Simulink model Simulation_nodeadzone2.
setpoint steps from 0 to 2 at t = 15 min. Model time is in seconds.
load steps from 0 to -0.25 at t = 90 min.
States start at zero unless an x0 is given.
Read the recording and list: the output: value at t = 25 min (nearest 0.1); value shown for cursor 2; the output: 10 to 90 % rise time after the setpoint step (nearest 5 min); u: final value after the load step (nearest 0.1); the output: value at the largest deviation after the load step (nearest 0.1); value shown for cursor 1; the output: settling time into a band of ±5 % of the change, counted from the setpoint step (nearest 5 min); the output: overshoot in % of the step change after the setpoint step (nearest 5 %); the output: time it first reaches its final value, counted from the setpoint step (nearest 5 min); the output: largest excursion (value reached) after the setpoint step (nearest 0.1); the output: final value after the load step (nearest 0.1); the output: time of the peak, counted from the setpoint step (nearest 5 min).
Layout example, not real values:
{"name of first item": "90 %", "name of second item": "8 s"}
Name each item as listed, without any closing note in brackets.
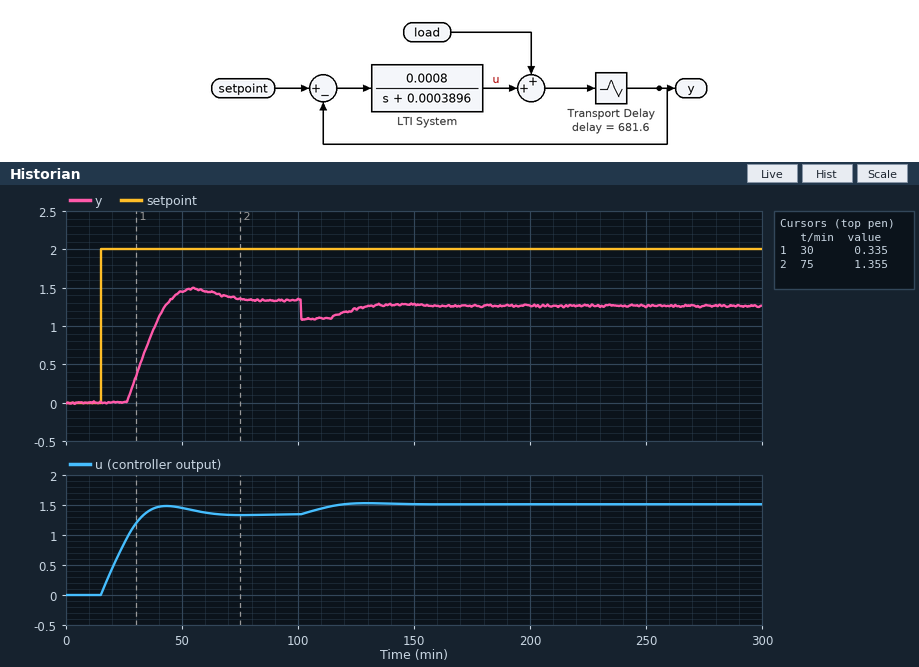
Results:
{"the output: value at t = 25 min": "0.0", "value shown for cursor 2": "1.355", "the output: 10 to 90 % rise time after the setpoint step": "15 min", "u: final value after the load step": "1.5", "the output: value at the largest deviation after the load step": "1.1", "value shown for cursor 1": "0.335", "the output: settling time into a band of ±5 % of the change, counted from the setpoint step": "50 min", "the output: overshoot in % of the step change after the setpoint step": "10 %", "the output: time it first reaches its final value, counted from the setpoint step": "30 min", "the output: largest excursion (value reached) after the setpoint step": "1.5", "the output: final value after the load step": "1.3", "the output: time of the peak, counted from the setpoint step": "40 min"}
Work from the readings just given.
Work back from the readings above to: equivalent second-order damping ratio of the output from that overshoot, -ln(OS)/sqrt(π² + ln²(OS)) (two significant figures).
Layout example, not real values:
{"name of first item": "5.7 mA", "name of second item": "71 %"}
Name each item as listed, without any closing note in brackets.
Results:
{"equivalent second-order damping ratio of the output from that overshoot, -ln(OS)/sqrt(π² + ln²(OS))": "0.59"}
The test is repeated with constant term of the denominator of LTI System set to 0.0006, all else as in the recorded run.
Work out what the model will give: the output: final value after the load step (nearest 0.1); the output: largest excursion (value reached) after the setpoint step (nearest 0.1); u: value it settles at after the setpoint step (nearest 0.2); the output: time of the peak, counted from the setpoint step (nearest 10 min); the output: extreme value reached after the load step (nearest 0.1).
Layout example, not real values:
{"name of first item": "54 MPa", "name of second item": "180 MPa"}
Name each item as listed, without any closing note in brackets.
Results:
{"the output: final value after the load step": "1.0", "the output: largest excursion (value reached) after the setpoint step": "1.3", "u: value it settles at after the setpoint step": "1.2", "the output: time of the peak, counted from the setpoint step": "40 min", "the output: extreme value reached after the load step": "0.9"}
